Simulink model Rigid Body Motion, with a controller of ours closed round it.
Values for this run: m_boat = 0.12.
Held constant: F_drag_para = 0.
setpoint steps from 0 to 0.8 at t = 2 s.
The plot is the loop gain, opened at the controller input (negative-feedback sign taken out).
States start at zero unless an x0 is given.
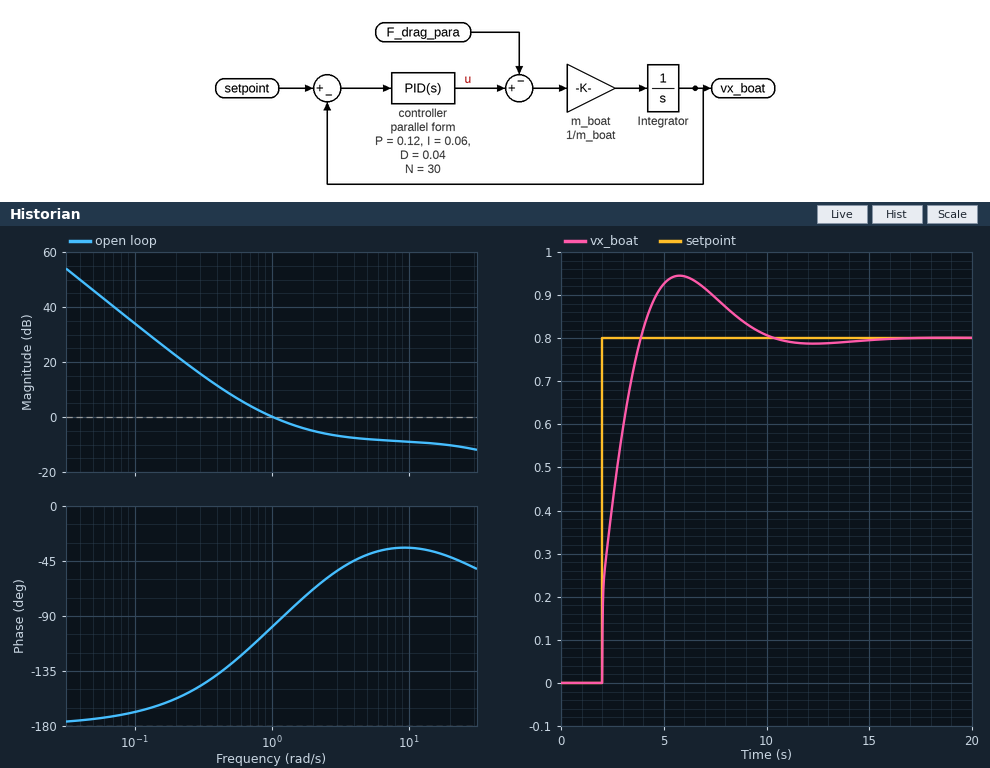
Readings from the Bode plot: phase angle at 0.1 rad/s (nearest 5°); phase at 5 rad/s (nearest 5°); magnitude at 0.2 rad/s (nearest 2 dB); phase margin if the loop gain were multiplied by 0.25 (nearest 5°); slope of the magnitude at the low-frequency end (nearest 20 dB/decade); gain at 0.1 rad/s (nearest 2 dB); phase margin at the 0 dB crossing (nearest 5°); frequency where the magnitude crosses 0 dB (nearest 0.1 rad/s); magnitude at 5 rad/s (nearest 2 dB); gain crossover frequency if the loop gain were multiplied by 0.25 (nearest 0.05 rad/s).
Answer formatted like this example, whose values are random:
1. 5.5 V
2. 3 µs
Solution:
1. -170°
2. -40°
3. 22 dB
4. 40°
5. -40 dB/decade
6. 34 dB
7. 80°
8. 1.0 rad/s
9. -8 dB
10. 0.40 rad/s
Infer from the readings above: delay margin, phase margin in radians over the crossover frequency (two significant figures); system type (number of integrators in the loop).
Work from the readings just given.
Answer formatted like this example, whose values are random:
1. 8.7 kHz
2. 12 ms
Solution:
1. 1.4 s
2. 2
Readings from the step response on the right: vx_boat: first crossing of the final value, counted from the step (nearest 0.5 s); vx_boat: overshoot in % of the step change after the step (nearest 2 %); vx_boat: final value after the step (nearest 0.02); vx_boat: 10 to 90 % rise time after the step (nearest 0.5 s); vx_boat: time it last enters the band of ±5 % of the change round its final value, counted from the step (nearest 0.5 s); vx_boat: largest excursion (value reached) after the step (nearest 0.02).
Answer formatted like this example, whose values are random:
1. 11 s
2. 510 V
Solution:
1. 2.0 s
2. 18 %
3. 0.80
4. 1.5 s
5. 7.0 s
6. 0.94
